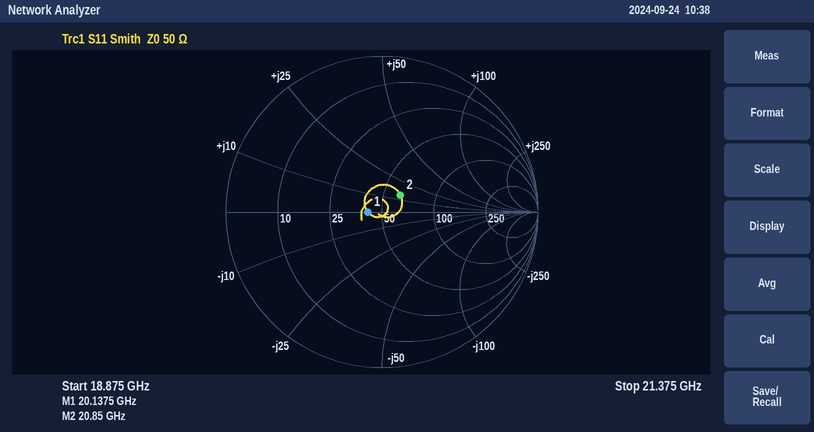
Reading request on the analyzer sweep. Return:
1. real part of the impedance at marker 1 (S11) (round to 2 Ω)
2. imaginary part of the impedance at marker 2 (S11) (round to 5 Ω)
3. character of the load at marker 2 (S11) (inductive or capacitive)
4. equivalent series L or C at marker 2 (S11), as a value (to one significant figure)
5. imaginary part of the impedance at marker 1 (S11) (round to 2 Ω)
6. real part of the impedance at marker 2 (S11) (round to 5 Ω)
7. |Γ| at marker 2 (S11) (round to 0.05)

42 Ω
+15 Ω
inductive
100 pH
0 Ω
60 Ω
0.15
